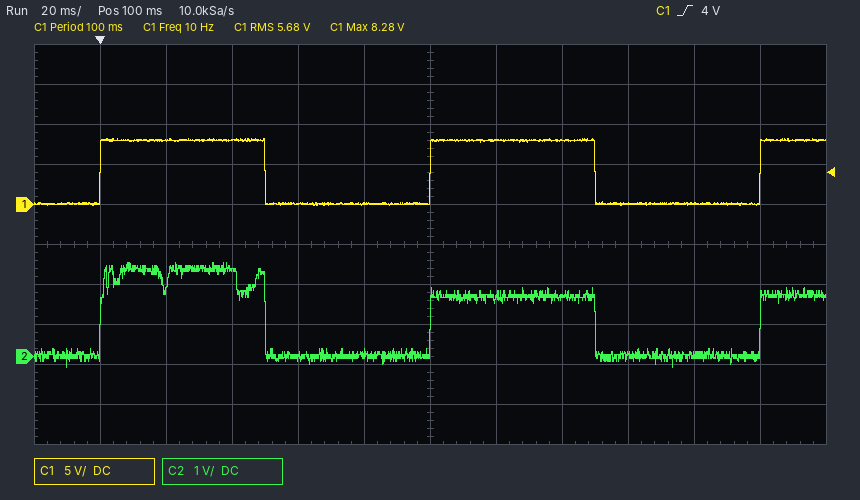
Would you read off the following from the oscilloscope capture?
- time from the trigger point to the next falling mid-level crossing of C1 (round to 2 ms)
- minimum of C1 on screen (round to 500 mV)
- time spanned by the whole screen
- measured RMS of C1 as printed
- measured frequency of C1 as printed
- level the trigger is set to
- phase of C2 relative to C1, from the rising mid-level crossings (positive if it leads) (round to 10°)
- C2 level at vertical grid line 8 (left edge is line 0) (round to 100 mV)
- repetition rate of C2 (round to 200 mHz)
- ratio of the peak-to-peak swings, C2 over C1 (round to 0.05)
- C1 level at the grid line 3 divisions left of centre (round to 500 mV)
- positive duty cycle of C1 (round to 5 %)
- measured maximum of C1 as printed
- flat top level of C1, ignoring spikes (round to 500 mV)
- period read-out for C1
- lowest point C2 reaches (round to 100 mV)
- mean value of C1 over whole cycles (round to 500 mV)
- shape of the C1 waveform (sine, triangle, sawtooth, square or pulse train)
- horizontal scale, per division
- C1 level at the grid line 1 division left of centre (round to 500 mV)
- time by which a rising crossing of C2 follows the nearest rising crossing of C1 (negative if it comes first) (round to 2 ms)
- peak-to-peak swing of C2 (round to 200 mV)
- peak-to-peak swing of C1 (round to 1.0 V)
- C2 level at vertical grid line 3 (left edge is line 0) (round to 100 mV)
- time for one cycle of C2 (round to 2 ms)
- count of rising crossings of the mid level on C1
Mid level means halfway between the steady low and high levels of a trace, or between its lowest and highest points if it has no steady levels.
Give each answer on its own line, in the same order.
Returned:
50 ms
0.0 V
240 ms
5.68 V
10 Hz
4 V
0°
1.5 V
10.0 Hz
0.30
8.0 V
50 %
8.28 V
8.0 V
100 ms
-300 mV
4.0 V
square
20 ms
0.0 V
0 ms
2.6 V
8.0 V
2.2 V
100 ms
3
